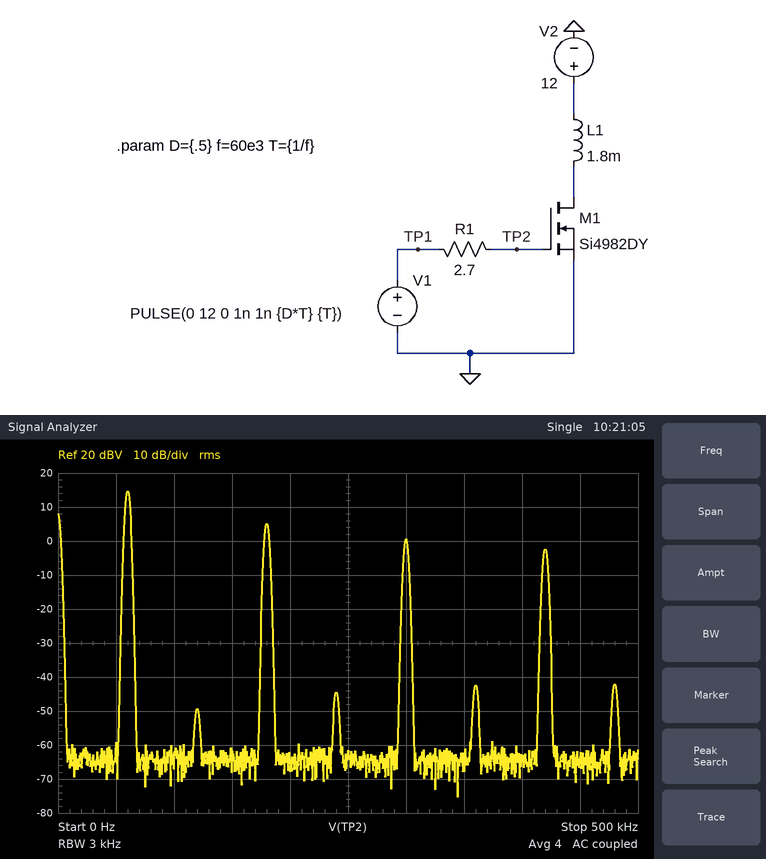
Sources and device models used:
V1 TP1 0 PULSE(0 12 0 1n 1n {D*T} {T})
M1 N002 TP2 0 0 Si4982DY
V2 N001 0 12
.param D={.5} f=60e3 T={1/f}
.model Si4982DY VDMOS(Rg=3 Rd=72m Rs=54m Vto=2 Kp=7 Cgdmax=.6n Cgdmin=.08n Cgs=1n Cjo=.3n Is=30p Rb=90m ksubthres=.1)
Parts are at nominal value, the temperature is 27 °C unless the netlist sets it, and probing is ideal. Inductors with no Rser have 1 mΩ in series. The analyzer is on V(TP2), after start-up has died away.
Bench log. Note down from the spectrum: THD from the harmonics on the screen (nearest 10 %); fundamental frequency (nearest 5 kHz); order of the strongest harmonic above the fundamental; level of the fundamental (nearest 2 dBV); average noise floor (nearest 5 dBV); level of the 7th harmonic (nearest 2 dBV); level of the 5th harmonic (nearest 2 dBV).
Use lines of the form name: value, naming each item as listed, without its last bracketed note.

THD from the harmonics on the screen: 40 %
fundamental frequency: 60 kHz
order of the strongest harmonic above the fundamental: 3
level of the fundamental: 14 dBV
average noise floor: -65 dBV
level of the 7th harmonic: -2 dBV
level of the 5th harmonic: 0 dBV
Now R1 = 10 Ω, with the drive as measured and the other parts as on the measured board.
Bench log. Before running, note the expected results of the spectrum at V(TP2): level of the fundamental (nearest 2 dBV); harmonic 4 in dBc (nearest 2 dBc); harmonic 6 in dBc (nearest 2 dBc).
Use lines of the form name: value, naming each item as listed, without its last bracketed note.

level of the fundamental: 14 dBV
harmonic 4 in dBc: -48 dBc
harmonic 6 in dBc: -46 dBc
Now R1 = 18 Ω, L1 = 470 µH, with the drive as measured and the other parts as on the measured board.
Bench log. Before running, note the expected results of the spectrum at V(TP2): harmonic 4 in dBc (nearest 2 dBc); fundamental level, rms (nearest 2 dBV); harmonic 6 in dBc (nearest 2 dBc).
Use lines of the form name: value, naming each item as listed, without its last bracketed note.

harmonic 4 in dBc: -42 dBc
fundamental level, rms: 14 dBV
harmonic 6 in dBc: -40 dBc
